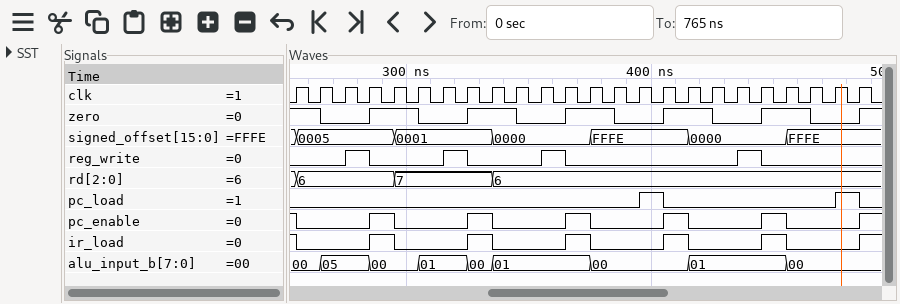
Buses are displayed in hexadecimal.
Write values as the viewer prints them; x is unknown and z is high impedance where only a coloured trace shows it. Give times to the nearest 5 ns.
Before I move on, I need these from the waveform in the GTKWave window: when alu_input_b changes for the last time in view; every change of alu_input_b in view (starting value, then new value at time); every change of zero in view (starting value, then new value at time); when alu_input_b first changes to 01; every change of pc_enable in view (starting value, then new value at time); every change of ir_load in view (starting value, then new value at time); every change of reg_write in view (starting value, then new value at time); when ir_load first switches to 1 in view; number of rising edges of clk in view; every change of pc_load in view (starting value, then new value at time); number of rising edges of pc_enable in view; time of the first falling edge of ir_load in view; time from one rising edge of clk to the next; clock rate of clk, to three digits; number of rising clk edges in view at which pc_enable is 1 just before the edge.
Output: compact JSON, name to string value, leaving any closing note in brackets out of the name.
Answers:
{"when alu_input_b changes for the last time in view": "455 ns", "every change of alu_input_b in view": "00, 05 at 265 ns, 00 at 285 ns, 01 at 305 ns, 00 at 325 ns, 01 at 335 ns, 00 at 375 ns, 01 at 415 ns, 00 at 455 ns", "every change of zero in view": "1, 0 at 265 ns, 1 at 285 ns, 0 at 305 ns, 1 at 325 ns, 0 at 345 ns, 1 at 365 ns, 0 at 385 ns, 1 at 405 ns, 0 at 425 ns, 1 at 445 ns, 0 at 465 ns, 1 at 485 ns", "when alu_input_b first changes to 01": "305 ns", "every change of pc_enable in view": "1, 0 at 255 ns, 1 at 285 ns, 0 at 295 ns, 1 at 325 ns, 0 at 335 ns, 1 at 365 ns, 0 at 375 ns, 1 at 405 ns, 0 at 415 ns, 1 at 445 ns, 0 at 455 ns, 1 at 485 ns", "every change of ir_load in view": "1, 0 at 255 ns, 1 at 285 ns, 0 at 295 ns, 1 at 325 ns, 0 at 335 ns, 1 at 365 ns, 0 at 375 ns, 1 at 405 ns, 0 at 415 ns, 1 at 445 ns, 0 at 455 ns, 1 at 485 ns", "every change of reg_write in view": "0, 1 at 275 ns, 0 at 285 ns, 1 at 315 ns, 0 at 325 ns, 1 at 355 ns, 0 at 365 ns, 1 at 435 ns, 0 at 445 ns", "when ir_load first switches to 1 in view": "285 ns", "number of rising edges of clk in view": "24", "every change of pc_load in view": "0, 1 at 395 ns, 0 at 405 ns, 1 at 475 ns, 0 at 485 ns", "number of rising edges of pc_enable in view": "6", "time of the first falling edge of ir_load in view": "255 ns", "time from one rising edge of clk to the next": "10 ns", "clock rate of clk, to three digits": "100 MHz", "number of rising clk edges in view at which pc_enable is 1 just before the edge": "6"}
